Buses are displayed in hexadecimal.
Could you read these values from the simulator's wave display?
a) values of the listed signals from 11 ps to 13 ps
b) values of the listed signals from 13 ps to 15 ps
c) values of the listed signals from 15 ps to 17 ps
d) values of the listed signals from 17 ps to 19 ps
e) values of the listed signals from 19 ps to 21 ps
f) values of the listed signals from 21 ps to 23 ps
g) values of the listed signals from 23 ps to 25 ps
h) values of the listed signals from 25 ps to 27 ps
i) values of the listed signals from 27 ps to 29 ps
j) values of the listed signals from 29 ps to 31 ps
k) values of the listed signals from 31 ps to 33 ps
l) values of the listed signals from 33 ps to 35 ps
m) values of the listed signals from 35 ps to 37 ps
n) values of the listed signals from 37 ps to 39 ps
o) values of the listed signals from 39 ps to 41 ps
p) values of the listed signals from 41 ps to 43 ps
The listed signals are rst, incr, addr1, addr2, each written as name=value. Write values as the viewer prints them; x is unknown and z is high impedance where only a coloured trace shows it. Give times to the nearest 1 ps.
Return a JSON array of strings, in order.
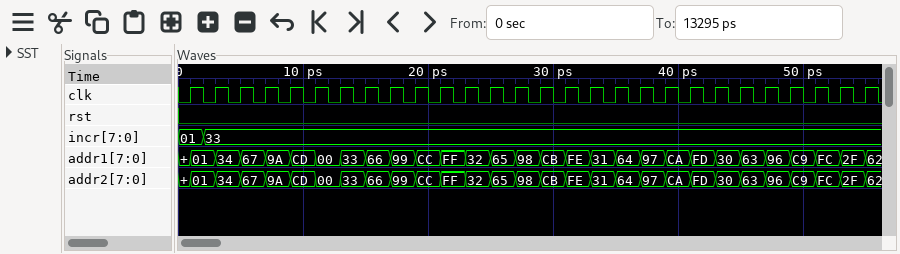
["rst=0, incr=33, addr1=00, addr2=00", "rst=0, incr=33, addr1=33, addr2=33", "rst=0, incr=33, addr1=66, addr2=66", "rst=0, incr=33, addr1=99, addr2=99", "rst=0, incr=33, addr1=CC, addr2=CC", "rst=0, incr=33, addr1=FF, addr2=FF", "rst=0, incr=33, addr1=32, addr2=32", "rst=0, incr=33, addr1=65, addr2=65", "rst=0, incr=33, addr1=98, addr2=98", "rst=0, incr=33, addr1=CB, addr2=CB", "rst=0, incr=33, addr1=FE, addr2=FE", "rst=0, incr=33, addr1=31, addr2=31", "rst=0, incr=33, addr1=64, addr2=64", "rst=0, incr=33, addr1=97, addr2=97", "rst=0, incr=33, addr1=CA, addr2=CA", "rst=0, incr=33, addr1=FD, addr2=FD"]
